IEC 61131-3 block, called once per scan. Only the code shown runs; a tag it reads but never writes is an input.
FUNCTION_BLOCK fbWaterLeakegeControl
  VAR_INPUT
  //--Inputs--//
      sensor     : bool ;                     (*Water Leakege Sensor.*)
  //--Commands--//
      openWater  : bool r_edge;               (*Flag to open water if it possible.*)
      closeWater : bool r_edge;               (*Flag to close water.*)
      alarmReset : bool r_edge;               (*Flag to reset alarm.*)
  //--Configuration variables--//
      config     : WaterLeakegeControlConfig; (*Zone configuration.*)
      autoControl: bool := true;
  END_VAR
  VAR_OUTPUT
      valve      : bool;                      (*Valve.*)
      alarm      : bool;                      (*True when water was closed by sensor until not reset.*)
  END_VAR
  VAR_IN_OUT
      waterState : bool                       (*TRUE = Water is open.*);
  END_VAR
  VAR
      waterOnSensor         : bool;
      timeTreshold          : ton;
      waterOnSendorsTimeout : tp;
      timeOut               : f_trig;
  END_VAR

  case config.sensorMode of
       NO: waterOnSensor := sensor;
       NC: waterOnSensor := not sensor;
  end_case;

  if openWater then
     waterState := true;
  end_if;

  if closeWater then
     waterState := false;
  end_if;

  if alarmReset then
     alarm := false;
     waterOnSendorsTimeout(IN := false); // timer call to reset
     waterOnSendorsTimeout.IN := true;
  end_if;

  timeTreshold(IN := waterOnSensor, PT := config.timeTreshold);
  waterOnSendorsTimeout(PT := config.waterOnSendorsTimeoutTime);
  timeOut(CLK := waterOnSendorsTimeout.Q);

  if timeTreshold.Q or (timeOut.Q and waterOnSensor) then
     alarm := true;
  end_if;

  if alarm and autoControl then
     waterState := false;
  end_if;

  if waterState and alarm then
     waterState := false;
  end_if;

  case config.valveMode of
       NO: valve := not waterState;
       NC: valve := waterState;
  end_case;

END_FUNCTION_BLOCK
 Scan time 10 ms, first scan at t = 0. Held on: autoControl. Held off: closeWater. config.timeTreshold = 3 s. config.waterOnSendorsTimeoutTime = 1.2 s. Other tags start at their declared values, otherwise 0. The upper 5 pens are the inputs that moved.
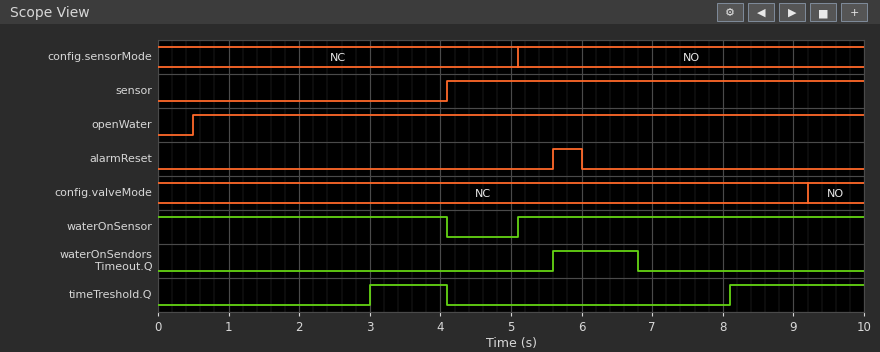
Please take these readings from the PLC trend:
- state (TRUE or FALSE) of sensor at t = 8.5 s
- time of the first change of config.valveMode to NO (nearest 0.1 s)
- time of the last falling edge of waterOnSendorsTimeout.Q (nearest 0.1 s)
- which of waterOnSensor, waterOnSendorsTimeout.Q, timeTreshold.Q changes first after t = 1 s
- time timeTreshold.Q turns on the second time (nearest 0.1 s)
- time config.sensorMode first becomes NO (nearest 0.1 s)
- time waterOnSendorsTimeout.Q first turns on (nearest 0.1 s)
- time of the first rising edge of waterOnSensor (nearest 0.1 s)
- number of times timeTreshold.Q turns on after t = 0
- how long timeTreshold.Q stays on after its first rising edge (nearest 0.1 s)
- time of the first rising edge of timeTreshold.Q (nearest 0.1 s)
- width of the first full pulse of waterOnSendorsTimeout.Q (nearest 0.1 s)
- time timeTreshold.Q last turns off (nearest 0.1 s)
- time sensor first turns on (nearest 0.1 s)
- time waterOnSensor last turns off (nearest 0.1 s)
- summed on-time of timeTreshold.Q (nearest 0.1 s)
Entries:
TRUE
9.2 s
6.8 s
timeTreshold.Q
8.1 s
5.1 s
5.6 s
5.1 s
2
1.1 s
3.0 s
1.2 s
4.1 s
4.1 s
4.1 s
3.0 s
